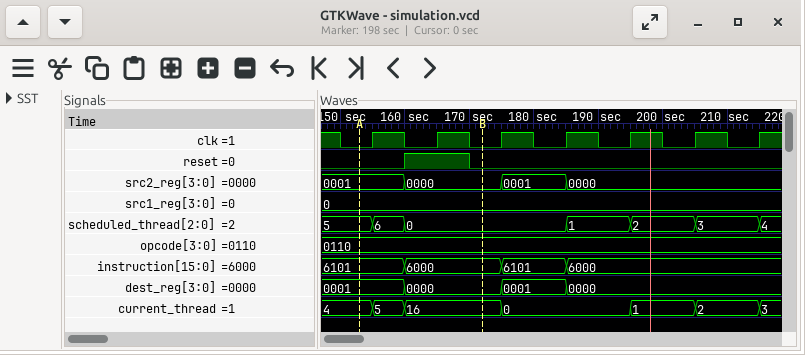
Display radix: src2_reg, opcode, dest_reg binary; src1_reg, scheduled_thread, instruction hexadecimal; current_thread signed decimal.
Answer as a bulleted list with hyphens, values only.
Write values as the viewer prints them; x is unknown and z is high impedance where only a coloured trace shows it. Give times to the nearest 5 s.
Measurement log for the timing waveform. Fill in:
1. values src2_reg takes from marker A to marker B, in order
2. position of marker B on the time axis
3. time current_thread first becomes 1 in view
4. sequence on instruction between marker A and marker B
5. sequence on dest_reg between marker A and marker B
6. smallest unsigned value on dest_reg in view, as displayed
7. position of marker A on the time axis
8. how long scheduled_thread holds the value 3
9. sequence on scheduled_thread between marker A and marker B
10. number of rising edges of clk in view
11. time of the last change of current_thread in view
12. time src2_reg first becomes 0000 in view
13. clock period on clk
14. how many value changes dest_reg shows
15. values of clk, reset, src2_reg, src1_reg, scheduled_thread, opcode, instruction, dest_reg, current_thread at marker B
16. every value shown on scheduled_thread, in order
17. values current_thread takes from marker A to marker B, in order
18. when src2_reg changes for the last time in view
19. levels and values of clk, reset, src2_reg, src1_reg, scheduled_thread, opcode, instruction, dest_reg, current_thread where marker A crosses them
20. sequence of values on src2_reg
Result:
- 0001, 0000
- 170 s
- 195 s
- 6101, 6000
- 0001, 0000
- 0000
- 155 s
- 10 s
- 5, 6, 0
- 7
- 215 s
- 160 s
- 10 s
- 3
- clk=0, reset=0, src2_reg=0000, src1_reg=0, scheduled_thread=0, opcode=0110, instruction=6000, dest_reg=0000, current_thread=16
- 5, 6, 0, 1, 2, 3, 4
- 4, 5, 16
- 185 s
- clk=0, reset=0, src2_reg=0001, src1_reg=0, scheduled_thread=5, opcode=0110, instruction=6101, dest_reg=0001, current_thread=4
- 0001, 0000, 0001, 0000
